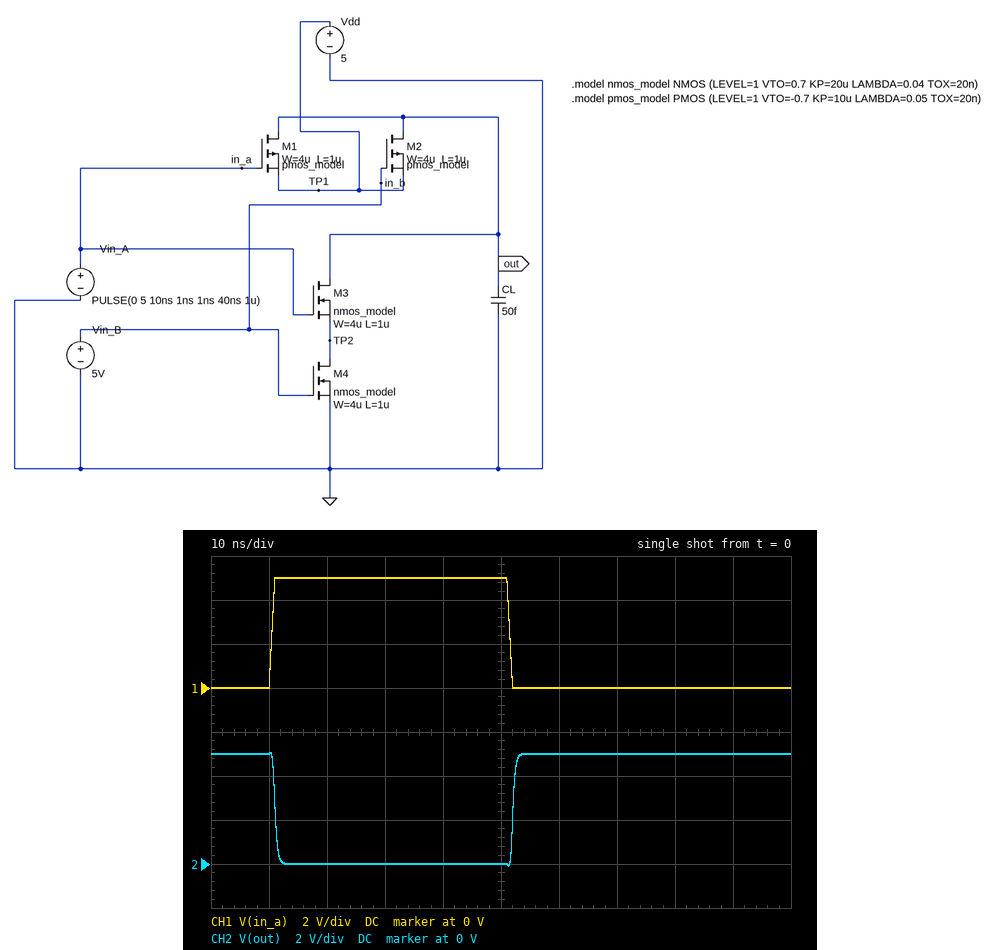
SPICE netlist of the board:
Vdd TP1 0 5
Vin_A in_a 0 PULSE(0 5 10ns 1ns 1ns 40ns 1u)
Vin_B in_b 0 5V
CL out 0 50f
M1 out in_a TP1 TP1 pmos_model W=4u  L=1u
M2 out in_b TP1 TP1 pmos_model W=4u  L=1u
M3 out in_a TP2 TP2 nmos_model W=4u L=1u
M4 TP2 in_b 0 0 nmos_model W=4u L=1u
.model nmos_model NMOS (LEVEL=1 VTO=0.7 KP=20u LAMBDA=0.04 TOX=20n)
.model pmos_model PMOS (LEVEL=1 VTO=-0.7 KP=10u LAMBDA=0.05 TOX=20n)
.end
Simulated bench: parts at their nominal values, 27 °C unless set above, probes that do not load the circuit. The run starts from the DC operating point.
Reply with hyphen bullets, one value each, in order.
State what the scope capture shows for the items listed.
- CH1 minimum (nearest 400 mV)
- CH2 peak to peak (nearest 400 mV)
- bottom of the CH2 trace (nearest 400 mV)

- 0 V
- 5.2 V
- 0 V
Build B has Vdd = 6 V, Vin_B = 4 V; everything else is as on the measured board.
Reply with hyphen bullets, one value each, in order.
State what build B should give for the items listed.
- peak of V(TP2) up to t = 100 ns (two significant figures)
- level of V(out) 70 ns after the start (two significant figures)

- 1.6 V
- 6.0 V
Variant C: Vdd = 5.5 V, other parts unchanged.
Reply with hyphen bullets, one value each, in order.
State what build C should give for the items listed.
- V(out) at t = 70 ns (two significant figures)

- 5.5 V
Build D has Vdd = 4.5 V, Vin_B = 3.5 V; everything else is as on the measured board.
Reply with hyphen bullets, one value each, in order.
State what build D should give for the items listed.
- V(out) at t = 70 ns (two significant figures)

- 4.5 V
